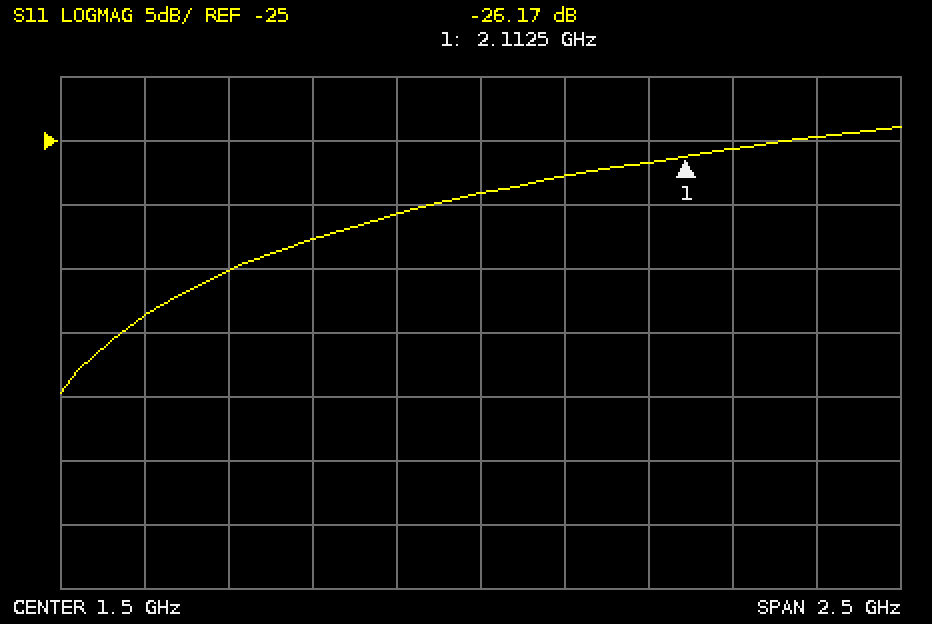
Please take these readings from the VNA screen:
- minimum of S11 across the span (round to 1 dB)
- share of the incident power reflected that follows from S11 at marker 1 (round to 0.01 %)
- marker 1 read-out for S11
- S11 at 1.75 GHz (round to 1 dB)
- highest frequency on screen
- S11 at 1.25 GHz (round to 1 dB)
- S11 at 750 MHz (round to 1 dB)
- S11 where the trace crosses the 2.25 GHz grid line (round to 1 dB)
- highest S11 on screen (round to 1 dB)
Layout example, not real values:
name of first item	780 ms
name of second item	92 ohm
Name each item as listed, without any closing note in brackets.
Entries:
minimum of S11 across the span	-45 dB
share of the incident power reflected that follows from S11 at marker 1	0.24 %
marker 1 read-out for S11	-26.17 dB
S11 at 1.75 GHz	-28 dB
highest frequency on screen	2.75 GHz
S11 at 1.25 GHz	-31 dB
S11 at 750 MHz	-35 dB
S11 where the trace crosses the 2.25 GHz grid line	-26 dB
highest S11 on screen	-24 dB
